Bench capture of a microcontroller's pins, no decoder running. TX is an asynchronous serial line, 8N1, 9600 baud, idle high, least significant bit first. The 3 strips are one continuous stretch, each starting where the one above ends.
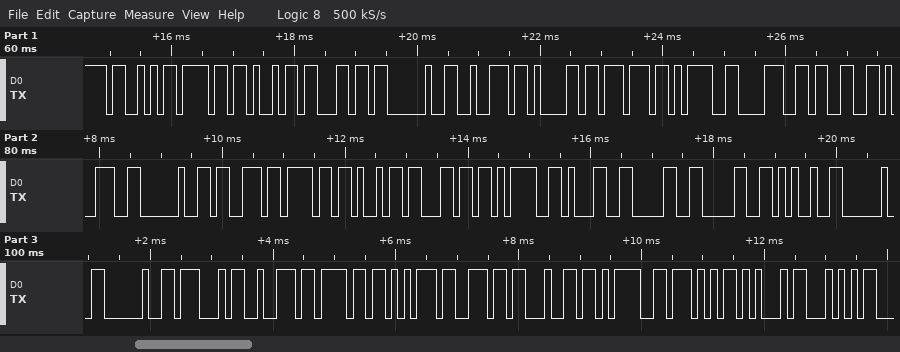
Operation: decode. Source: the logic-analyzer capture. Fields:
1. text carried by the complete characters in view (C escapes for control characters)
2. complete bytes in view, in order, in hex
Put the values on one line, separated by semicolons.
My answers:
"Soil raw=839 soil=100%  Ground=WET"; 53 6F 69 6C 20 72 61 77 3D 38 33 39 20 73 6F 69 6C 3D 31 30 30 25 20 20 47 72 6F 75 6E 64 3D 57 45 54
